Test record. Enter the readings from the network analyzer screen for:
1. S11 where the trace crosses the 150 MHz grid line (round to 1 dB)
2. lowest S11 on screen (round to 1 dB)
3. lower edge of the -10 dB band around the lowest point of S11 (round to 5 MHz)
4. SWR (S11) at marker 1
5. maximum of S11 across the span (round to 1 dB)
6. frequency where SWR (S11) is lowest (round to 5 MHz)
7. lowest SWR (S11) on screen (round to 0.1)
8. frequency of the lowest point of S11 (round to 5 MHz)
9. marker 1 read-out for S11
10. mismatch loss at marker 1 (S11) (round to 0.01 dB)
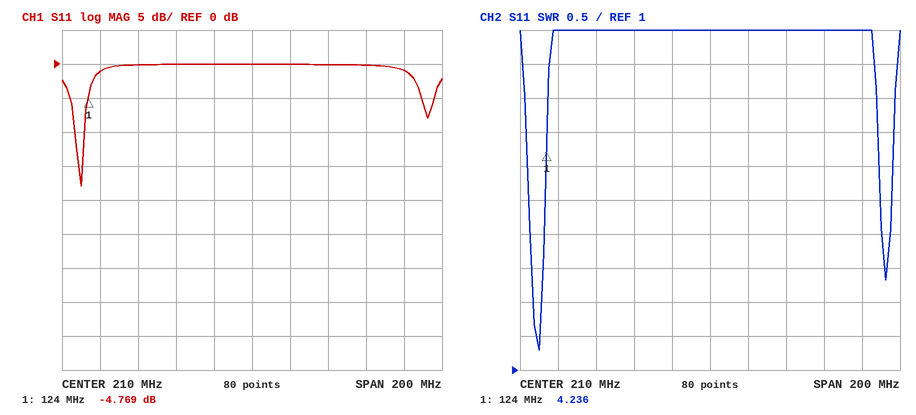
0 dB
-18 dB
115 MHz
4.236
0 dB
120 MHz
1.3
120 MHz
-4.769 dB
1.76 dB
